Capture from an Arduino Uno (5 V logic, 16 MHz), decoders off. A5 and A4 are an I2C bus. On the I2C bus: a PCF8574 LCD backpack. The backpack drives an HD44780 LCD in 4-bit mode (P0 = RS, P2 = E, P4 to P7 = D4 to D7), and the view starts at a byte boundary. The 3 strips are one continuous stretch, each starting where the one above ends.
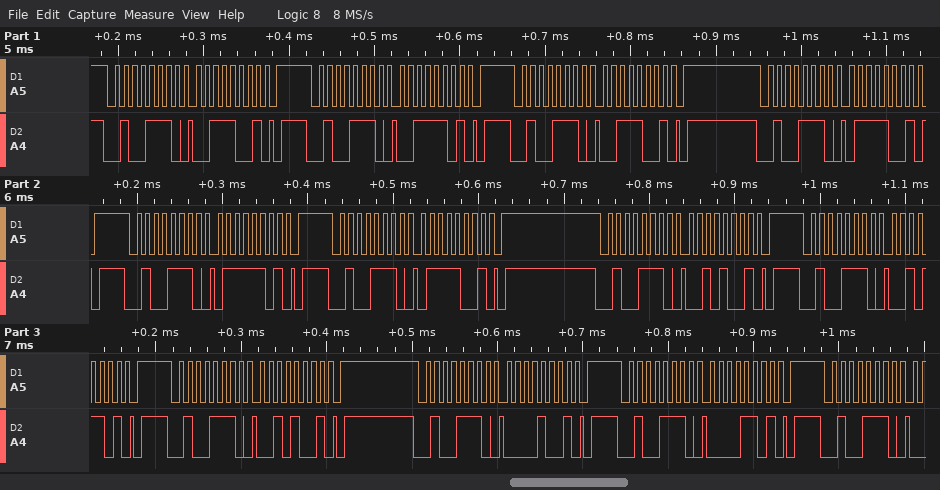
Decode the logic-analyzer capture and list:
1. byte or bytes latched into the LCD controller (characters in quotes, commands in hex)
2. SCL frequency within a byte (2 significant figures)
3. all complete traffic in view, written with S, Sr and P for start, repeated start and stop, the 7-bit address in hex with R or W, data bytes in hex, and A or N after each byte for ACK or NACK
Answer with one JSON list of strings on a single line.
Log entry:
["'7'", "100 kHz", "S 27W A 39 A P S 27W A 3D A P S 27W A 39 A P S 27W A 79 A P S 27W A 7D A P S 27W A 79 A P S 27W A 29 A P S 27W A 2D A P S 27W A 29 A P S 27W A 09 A P S 27W A 0D A P S 27W A"]
